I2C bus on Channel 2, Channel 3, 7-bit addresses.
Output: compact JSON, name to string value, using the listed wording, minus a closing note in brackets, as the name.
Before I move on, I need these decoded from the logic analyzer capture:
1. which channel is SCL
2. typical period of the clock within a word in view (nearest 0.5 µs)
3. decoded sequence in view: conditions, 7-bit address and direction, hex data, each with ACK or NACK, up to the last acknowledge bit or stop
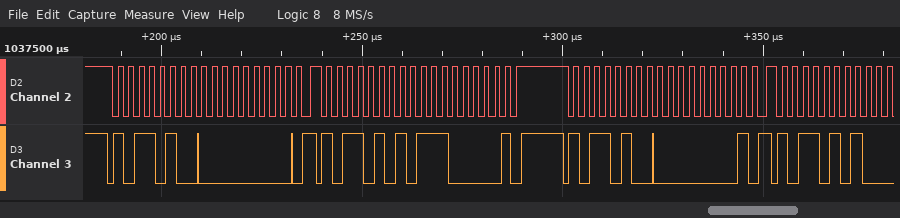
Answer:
{"which channel is SCL": "Channel 2", "typical period of the clock within a word in view": "2.5 µs", "decoded sequence in view: conditions, 7-bit address and direction, hex data, each with ACK or NACK, up to the last acknowledge bit or stop": "start, address 5A write ACK, 00 ACK, repeated start, address 5A read ACK, E0 NACK, stop, start, address 5A write ACK, 01 ACK, repeated start, address 5A read ACK"}
